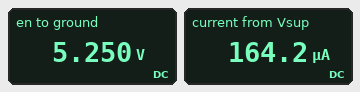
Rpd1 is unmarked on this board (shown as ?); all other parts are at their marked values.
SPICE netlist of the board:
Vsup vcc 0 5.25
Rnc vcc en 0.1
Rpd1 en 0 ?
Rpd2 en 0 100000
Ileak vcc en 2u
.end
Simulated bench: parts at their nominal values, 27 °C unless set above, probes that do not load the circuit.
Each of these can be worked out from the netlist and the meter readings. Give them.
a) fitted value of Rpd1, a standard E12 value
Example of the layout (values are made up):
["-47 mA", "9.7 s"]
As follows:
["47 kΩ"]
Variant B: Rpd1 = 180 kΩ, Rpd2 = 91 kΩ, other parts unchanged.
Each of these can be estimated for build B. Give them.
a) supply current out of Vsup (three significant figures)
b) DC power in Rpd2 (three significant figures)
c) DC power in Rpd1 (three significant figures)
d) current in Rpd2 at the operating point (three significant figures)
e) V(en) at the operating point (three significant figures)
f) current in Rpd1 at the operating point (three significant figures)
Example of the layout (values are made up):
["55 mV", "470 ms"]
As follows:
["86.9 µA", "303 µW", "153 µW", "57.7 µA", "5.25 V", "29.2 µA"]
